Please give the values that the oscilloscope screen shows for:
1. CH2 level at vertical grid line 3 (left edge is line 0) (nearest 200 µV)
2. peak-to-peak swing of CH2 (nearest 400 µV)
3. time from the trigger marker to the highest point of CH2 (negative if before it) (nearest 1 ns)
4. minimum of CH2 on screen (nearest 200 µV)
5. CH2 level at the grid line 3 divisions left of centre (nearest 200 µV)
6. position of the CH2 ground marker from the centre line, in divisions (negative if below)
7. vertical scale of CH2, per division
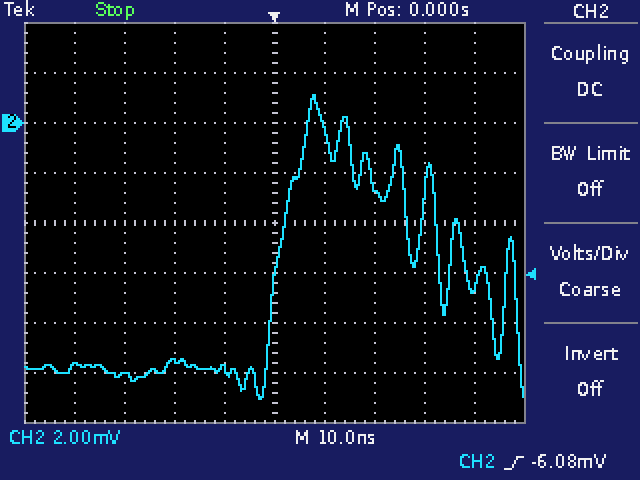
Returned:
-9.6 mV
12.0 mV
+8 ns
-11.0 mV
-10.0 mV
+2.0 div
2 mV
